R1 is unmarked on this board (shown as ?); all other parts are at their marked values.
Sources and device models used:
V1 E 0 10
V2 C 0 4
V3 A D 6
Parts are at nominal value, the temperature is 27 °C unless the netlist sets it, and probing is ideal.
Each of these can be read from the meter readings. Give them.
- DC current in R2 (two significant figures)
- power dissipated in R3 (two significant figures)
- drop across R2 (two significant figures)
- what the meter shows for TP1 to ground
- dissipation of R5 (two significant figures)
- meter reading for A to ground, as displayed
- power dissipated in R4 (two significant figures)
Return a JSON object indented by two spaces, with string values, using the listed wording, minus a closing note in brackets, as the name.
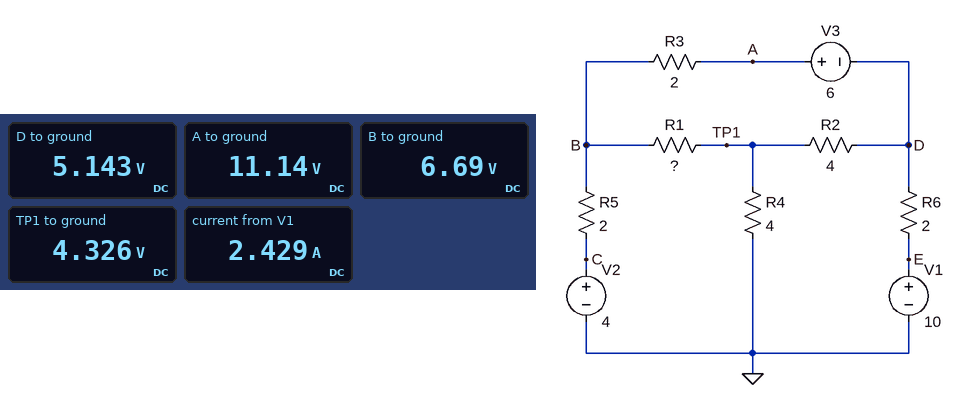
{
  "DC current in R2": "200 mA",
  "power dissipated in R3": "9.9 W",
  "drop across R2": "820 mV",
  "what the meter shows for TP1 to ground": "4.326 V",
  "dissipation of R5": "3.6 W",
  "meter reading for A to ground, as displayed": "11.14 V",
  "power dissipated in R4": "4.7 W"
}
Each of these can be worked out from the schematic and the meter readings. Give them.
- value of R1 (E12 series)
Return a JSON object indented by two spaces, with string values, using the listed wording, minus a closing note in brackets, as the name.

{
  "value of R1": "2.7 Ω"
}
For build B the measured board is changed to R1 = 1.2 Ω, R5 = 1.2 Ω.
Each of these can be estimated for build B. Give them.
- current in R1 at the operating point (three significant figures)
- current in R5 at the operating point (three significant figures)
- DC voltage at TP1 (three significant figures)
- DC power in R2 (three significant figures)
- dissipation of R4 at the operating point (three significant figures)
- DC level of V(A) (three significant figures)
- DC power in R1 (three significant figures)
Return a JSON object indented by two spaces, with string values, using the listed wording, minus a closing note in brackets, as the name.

{
  "current in R1 at the operating point": "1.05 A",
  "current in R5 at the operating point": "1.47 A",
  "DC voltage at TP1": "4.50 V",
  "DC power in R2": "22.9 mW",
  "dissipation of R4 at the operating point": "5.07 W",
  "DC level of V(A)": "10.8 V",
  "DC power in R1": "1.32 W"
}
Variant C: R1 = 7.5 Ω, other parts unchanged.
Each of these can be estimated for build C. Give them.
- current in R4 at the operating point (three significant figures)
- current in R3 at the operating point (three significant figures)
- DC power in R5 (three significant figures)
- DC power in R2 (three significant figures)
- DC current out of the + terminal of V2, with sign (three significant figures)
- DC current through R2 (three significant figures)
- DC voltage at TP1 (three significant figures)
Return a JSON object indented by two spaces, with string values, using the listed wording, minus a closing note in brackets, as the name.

{
  "current in R4 at the operating point": "881 mA",
  "current in R3 at the operating point": "2.02 A",
  "DC power in R5": "4.79 W",
  "DC power in R2": "655 mW",
  "DC current out of the + terminal of V2, with sign": "-1.55 A",
  "DC current through R2": "405 mA",
  "DC voltage at TP1": "3.52 V"
}
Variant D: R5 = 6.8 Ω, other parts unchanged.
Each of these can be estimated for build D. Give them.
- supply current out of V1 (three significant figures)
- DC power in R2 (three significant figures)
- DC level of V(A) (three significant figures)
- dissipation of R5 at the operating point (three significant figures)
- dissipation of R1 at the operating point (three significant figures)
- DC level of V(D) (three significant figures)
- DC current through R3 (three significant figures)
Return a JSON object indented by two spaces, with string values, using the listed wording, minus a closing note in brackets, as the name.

{
  "supply current out of V1": "1.98 A",
  "DC power in R2": "128 mW",
  "DC level of V(A)": "12.0 V",
  "dissipation of R5 at the operating point": "2.89 W",
  "dissipation of R1 at the operating point": "3.58 W",
  "DC level of V(D)": "6.04 V",
  "DC current through R3": "1.80 A"
}
